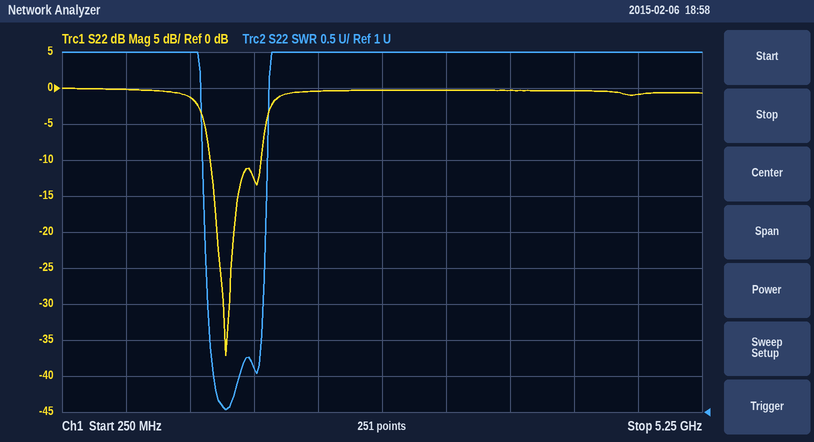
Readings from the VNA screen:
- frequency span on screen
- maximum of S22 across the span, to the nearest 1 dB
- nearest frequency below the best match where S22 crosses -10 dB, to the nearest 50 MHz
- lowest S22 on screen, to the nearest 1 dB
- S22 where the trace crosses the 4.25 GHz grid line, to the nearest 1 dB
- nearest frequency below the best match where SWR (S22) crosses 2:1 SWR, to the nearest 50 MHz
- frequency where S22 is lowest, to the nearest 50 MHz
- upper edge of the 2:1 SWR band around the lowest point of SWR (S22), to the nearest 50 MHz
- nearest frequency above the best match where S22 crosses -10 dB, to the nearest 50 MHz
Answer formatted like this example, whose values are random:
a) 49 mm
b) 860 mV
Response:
a) 5 GHz
b) 0 dB
c) 1.40 GHz
d) -37 dB
e) 0 dB
f) 1.40 GHz
g) 1.55 GHz
h) 1.80 GHz
i) 1.80 GHz
